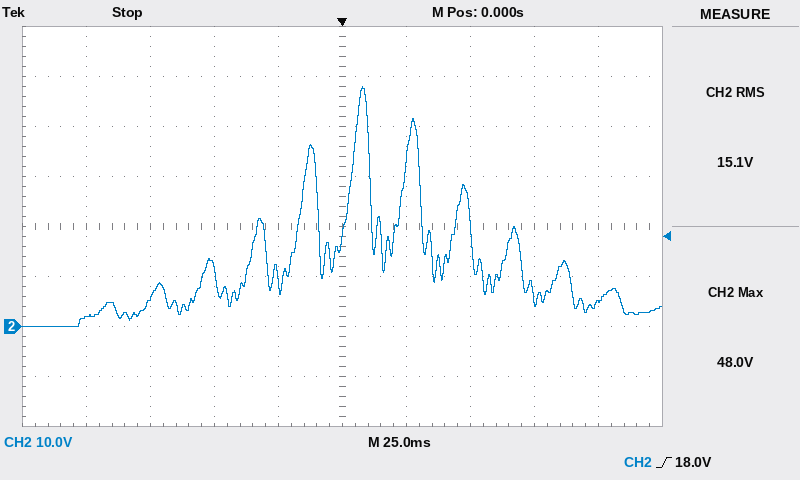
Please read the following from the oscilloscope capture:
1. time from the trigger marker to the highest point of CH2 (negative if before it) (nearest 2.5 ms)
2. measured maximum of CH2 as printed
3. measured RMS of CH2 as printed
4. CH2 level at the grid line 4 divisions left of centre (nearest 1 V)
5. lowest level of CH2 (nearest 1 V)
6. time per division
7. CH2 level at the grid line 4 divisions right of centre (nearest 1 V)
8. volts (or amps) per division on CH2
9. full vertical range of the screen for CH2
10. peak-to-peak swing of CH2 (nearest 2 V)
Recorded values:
+7.5 ms
48.0 V
15.1 V
2 V
0 V
25 ms
5 V
10 V
80 V
48 V
